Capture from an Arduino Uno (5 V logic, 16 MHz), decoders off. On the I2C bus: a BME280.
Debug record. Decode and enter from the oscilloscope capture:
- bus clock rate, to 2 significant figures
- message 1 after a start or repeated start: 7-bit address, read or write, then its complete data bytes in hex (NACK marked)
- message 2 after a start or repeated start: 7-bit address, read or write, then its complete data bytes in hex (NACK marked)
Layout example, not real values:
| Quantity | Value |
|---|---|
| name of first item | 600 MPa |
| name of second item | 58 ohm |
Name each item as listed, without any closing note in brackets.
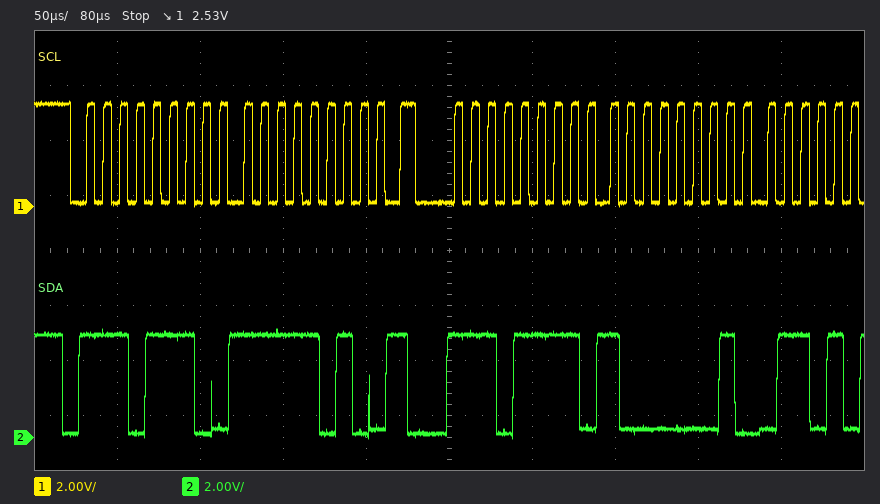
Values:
| Quantity | Value |
|---|---|
| bus clock rate, to 2 significant figures | 100 kHz |
| message 1 after a start or repeated start: 7-bit address, read or write, then its complete data bytes in hex | 0x77 write: FA |
| message 2 after a start or repeated start: 7-bit address, read or write, then its complete data bytes in hex | 0x77 read: 81 |
